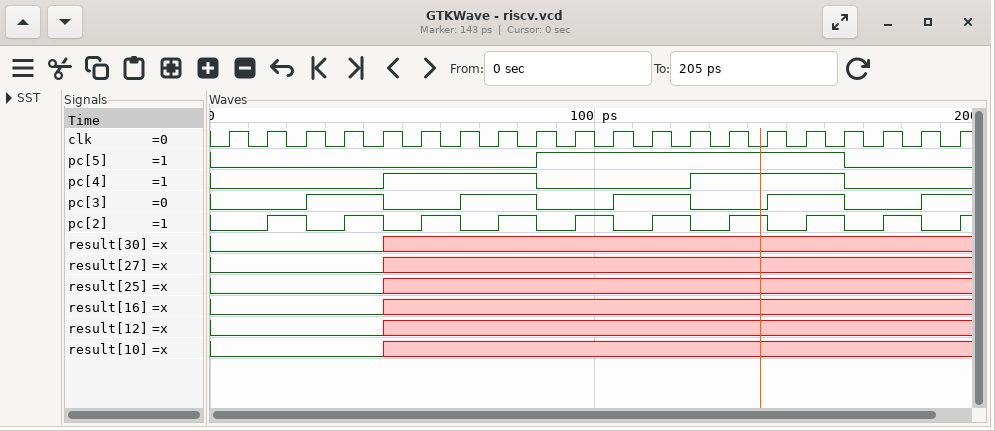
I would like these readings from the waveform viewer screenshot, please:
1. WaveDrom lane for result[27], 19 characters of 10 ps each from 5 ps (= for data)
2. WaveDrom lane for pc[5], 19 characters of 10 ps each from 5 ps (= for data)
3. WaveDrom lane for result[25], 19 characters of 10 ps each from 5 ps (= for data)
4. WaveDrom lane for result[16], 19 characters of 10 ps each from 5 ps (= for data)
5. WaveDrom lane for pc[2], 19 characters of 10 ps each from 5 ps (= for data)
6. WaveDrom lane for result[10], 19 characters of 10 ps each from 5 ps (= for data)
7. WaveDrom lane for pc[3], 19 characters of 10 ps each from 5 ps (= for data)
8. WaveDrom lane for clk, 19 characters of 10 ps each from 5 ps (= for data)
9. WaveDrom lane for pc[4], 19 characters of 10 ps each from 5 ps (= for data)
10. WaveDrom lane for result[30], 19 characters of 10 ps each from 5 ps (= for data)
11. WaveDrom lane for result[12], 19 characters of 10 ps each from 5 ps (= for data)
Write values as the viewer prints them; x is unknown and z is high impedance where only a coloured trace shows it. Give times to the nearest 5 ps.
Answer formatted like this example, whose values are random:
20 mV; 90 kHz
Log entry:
{name: 'result[27]', wave: '0...x..............'}; {name: 'pc[5]', wave: '0.......1.......0..'}; {name: 'result[25]', wave: '0...x..............'}; {name: 'result[16]', wave: '0...x..............'}; {name: 'pc[2]', wave: '0101010101010101010'}; {name: 'result[10]', wave: '0...x..............'}; {name: 'pc[3]', wave: '0.1.0.1.0.1.0.1.0.1'}; {name: 'clk', wave: 'p..................'}; {name: 'pc[4]', wave: '0...1...0...1...0..'}; {name: 'result[30]', wave: '0...x..............'}; {name: 'result[12]', wave: '0...x..............'}
